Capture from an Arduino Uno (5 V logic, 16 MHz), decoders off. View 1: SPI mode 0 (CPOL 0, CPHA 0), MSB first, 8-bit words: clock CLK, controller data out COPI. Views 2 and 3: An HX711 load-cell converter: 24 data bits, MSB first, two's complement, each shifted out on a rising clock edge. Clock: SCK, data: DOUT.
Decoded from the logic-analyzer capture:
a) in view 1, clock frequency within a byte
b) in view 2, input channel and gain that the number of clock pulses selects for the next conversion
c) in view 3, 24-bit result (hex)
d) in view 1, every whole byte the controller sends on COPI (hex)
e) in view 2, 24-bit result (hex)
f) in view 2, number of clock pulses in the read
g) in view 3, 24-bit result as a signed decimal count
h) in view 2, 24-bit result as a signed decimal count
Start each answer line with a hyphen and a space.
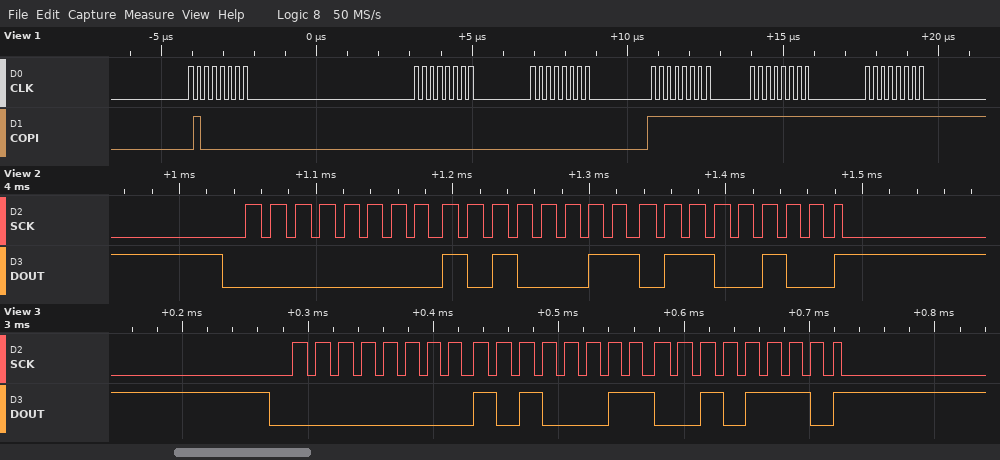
- 4 MHz
- channel A, gain 128
- 0x00A32E
- 40 00 00 FF FF FF
- 0x00A364
- 25
- 41774
- 41828
